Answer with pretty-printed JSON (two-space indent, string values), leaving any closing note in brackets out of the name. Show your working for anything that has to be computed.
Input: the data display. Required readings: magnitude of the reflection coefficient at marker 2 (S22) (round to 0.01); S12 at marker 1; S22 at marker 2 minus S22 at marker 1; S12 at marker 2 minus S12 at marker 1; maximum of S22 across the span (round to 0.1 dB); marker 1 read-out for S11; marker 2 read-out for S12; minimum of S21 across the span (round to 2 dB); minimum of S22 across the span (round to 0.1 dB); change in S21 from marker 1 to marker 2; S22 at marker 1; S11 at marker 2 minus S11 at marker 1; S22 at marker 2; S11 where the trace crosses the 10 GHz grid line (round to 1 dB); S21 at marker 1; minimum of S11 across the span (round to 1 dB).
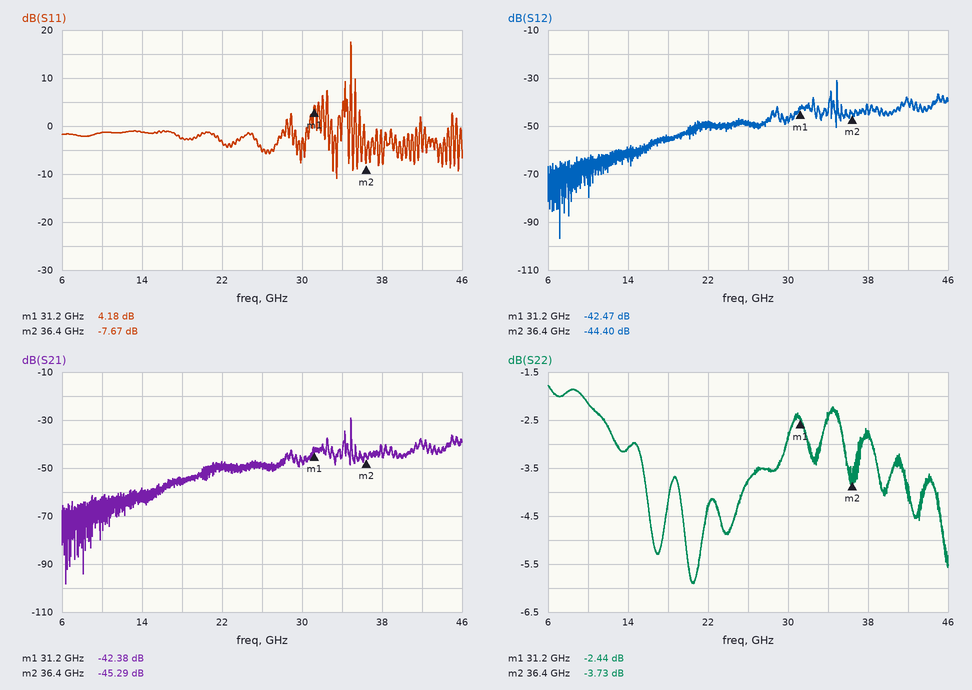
{
  "magnitude of the reflection coefficient at marker 2 (S22)": "10^(-3.73/20) ≈ 0.65",
  "S12 at marker 1": "-42.47 dB",
  "S22 at marker 2 minus S22 at marker 1": "-3.73 − (-2.44) = -1.29 dB",
  "S12 at marker 2 minus S12 at marker 1": "-44.4 − (-42.47) = -1.93 dB",
  "maximum of S22 across the span": "-1.8 dB",
  "marker 1 read-out for S11": "4.18 dB",
  "marker 2 read-out for S12": "-44.40 dB",
  "minimum of S21 across the span": "-98 dB",
  "minimum of S22 across the span": "-5.9 dB",
  "change in S21 from marker 1 to marker 2": "-45.29 − (-42.38) = -2.91 dB",
  "S22 at marker 1": "-2.44 dB",
  "S11 at marker 2 minus S11 at marker 1": "-7.67 − (4.18) = -11.85 dB",
  "S22 at marker 2": "-3.73 dB",
  "S11 where the trace crosses the 10 GHz grid line": "-1 dB",
  "S21 at marker 1": "-42.38 dB",
  "minimum of S11 across the span": "-11 dB"
}
